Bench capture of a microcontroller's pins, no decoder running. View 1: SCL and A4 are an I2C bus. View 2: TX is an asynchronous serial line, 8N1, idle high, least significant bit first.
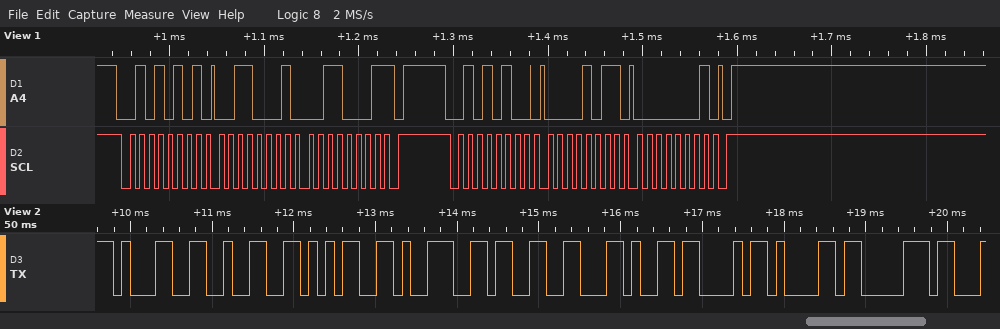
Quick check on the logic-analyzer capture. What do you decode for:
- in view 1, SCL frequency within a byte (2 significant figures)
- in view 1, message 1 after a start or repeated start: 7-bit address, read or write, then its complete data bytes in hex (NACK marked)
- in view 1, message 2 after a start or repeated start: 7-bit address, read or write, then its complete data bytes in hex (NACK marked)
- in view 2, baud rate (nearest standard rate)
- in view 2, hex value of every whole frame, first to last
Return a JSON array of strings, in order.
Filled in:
["100 kHz", "0x2A read: 31 31 NACK", "0x2A write: 0B 01", "9600 baud", "0x31 0x32 0x35 0x39 0x33 0x2C 0x43 0x61 0x70"]
